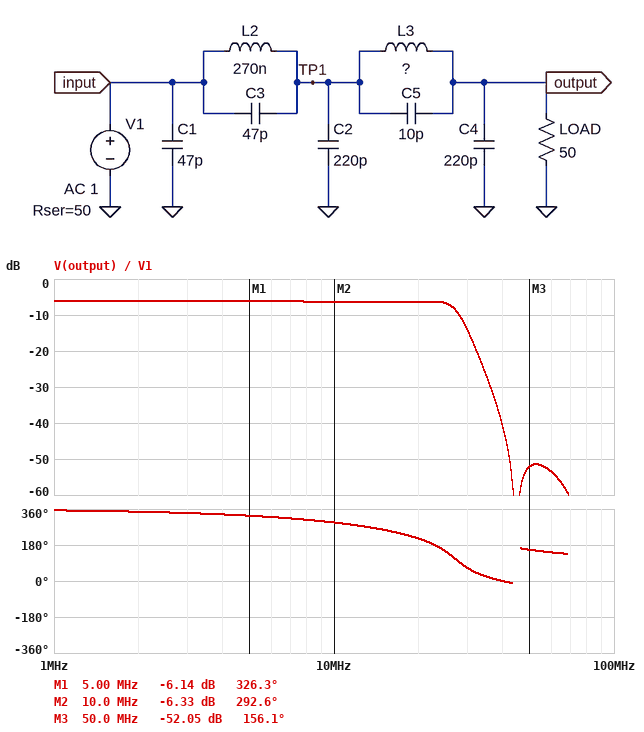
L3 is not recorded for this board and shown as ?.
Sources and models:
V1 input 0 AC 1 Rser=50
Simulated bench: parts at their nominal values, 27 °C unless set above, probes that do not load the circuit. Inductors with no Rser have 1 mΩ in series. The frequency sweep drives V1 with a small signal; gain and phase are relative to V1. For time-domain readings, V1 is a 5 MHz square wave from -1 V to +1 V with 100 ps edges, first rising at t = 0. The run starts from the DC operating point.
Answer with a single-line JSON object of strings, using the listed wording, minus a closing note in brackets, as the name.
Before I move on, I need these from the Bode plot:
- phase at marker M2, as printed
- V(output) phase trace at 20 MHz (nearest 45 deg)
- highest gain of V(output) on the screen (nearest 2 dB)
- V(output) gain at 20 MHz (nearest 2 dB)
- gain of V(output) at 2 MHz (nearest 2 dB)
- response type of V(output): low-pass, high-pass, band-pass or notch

{"phase at marker M2, as printed": "292.6 deg", "V(output) phase trace at 20 MHz": "225 deg", "highest gain of V(output) on the screen": "-6 dB", "V(output) gain at 20 MHz": "-6 dB", "gain of V(output) at 2 MHz": "-6 dB", "response type of V(output): low-pass, high-pass, band-pass or notch": "low-pass"}
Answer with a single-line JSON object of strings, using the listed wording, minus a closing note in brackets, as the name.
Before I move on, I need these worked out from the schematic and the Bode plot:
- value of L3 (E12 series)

{"value of L3": "390 nH"}
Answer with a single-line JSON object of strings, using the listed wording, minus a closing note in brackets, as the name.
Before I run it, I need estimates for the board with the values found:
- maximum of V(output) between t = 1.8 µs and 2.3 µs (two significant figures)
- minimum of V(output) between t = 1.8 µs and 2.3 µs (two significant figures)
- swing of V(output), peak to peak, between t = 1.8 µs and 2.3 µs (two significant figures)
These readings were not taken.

{"maximum of V(output) between t = 1.8 µs and 2.3 µs": "650 mV", "minimum of V(output) between t = 1.8 µs and 2.3 µs": "-650 mV", "swing of V(output), peak to peak, between t = 1.8 µs and 2.3 µs": "1.3 V"}
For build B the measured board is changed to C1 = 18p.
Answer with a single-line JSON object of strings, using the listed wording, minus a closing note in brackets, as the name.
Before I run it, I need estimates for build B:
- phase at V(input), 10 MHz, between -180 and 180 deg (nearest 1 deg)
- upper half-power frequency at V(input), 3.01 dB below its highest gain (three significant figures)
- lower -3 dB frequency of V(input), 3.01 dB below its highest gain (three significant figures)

{"phase at V(input), 10 MHz, between -180 and 180 deg": "6 deg", "upper half-power frequency at V(input), 3.01 dB below its highest gain": "72.7 MHz", "lower -3 dB frequency of V(input), 3.01 dB below its highest gain": "29.2 MHz"}
